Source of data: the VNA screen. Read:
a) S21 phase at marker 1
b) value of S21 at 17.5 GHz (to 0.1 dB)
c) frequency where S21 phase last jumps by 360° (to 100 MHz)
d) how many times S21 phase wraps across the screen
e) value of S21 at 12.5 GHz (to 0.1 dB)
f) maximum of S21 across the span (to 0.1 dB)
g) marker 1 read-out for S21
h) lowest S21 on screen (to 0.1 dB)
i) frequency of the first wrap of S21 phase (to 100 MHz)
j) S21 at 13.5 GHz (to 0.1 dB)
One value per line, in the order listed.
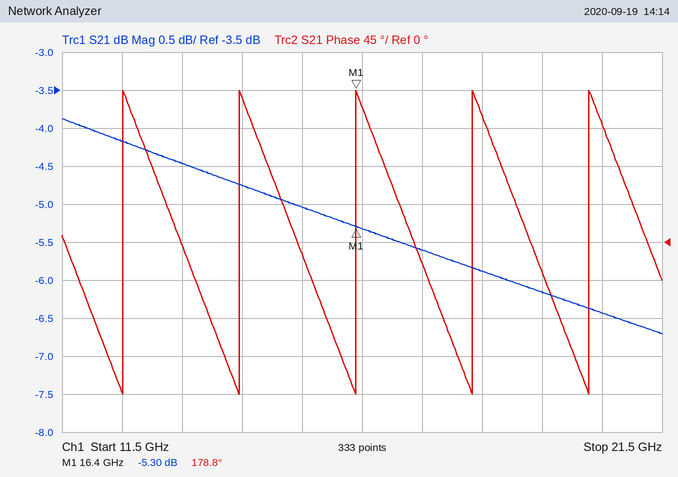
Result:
178.8°
-5.6 dB
20.3 GHz
5
-4.2 dB
-3.9 dB
-5.30 dB
-6.7 dB
12.5 GHz
-4.5 dB
